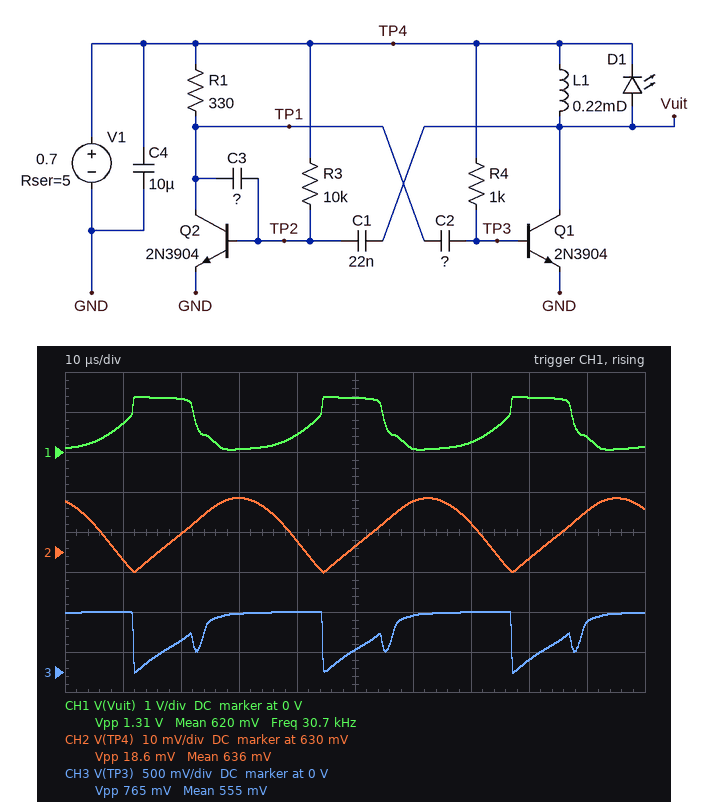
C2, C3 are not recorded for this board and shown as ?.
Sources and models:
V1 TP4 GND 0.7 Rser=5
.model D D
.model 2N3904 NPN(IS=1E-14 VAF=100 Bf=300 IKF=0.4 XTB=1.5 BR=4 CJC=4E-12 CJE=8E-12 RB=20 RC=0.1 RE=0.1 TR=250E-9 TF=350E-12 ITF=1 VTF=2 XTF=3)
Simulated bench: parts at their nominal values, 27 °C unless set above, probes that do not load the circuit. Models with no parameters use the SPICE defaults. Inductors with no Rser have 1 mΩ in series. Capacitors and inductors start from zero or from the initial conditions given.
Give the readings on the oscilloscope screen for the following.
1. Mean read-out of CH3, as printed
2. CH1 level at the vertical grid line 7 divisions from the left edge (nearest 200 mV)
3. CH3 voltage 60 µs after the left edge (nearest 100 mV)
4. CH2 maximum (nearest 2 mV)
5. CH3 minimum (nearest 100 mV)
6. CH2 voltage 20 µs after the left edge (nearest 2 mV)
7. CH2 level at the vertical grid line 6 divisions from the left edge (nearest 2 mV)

555 mV
200 mV
700 mV
644 mV
0 V
634 mV
642 mV
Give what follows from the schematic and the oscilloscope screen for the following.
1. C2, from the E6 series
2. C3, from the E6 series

10 nF
10 nF
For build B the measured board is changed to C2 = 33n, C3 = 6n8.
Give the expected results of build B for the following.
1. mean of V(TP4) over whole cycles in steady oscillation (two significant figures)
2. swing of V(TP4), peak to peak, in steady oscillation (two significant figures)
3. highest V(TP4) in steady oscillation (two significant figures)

620 mV
24 mV
630 mV
